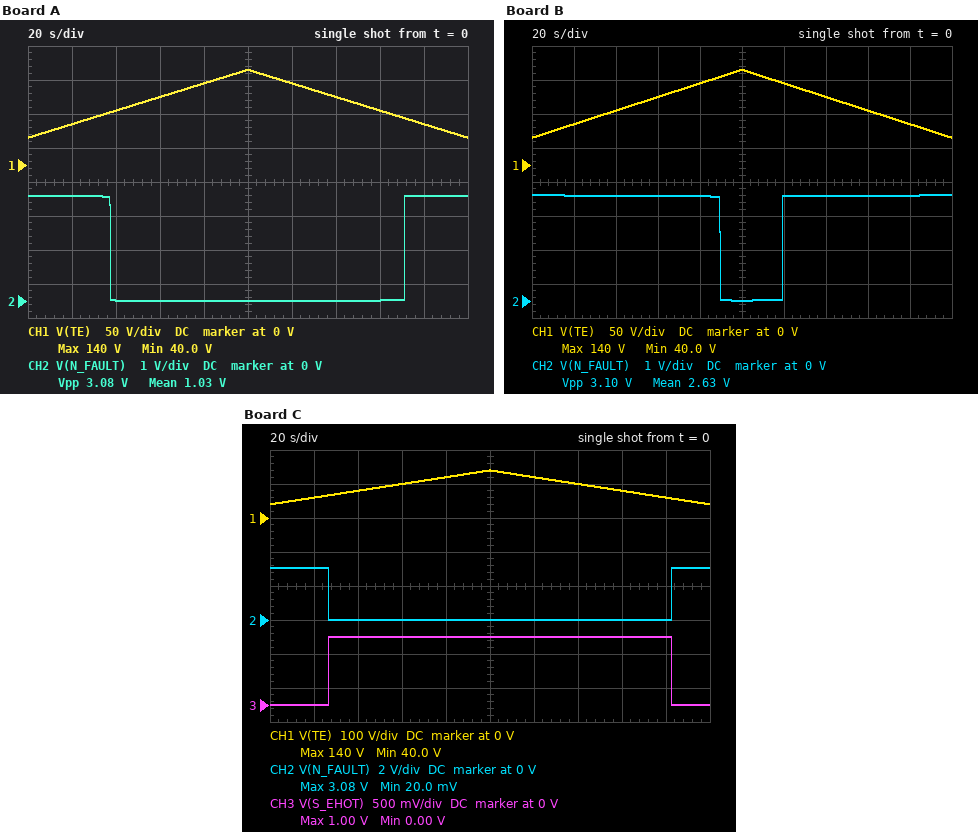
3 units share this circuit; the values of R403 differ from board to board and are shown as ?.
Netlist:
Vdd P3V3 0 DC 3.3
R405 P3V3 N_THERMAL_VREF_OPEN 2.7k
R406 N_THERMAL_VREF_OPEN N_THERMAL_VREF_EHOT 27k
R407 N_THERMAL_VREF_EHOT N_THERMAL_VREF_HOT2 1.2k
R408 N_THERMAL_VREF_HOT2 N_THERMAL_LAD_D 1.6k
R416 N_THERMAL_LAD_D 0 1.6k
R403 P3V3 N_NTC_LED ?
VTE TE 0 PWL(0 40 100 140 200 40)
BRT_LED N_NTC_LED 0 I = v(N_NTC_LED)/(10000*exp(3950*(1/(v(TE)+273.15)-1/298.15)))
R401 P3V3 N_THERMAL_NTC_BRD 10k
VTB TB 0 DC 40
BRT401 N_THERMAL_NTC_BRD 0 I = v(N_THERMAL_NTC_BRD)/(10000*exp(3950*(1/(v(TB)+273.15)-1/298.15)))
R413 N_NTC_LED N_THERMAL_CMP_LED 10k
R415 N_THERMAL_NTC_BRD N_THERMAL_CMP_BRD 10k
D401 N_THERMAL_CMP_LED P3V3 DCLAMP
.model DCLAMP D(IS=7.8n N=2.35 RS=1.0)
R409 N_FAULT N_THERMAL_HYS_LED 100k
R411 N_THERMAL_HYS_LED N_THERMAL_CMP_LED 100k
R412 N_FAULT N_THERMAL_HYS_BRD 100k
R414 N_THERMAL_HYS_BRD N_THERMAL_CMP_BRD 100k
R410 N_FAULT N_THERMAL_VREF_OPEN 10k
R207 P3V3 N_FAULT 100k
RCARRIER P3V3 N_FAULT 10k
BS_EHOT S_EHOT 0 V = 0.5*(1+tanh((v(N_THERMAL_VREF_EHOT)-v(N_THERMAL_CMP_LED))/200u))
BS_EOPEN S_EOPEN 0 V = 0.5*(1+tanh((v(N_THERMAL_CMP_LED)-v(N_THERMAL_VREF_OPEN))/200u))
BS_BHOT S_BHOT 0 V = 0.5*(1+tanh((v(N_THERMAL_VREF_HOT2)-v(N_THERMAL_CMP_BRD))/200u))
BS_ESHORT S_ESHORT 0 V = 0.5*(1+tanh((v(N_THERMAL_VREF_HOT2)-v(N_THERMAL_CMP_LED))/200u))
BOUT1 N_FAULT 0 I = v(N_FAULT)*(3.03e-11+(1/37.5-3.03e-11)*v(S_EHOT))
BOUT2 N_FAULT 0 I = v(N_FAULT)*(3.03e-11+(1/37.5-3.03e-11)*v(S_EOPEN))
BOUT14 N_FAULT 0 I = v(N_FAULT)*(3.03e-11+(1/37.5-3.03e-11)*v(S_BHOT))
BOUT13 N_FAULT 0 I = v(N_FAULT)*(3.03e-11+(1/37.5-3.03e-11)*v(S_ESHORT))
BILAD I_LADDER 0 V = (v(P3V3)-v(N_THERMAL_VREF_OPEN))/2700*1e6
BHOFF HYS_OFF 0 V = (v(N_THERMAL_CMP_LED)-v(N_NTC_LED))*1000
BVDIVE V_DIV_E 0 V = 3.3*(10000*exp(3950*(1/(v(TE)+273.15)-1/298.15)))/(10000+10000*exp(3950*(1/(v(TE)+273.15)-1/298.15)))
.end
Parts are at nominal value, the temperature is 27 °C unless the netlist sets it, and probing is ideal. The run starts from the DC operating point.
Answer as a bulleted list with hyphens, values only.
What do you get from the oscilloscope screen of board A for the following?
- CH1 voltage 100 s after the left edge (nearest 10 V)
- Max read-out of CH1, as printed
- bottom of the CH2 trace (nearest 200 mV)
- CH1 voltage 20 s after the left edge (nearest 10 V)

- 140 V
- 140 V
- 0 V
- 60 V
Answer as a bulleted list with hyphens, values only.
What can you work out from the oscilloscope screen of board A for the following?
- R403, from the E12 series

- 15 kΩ
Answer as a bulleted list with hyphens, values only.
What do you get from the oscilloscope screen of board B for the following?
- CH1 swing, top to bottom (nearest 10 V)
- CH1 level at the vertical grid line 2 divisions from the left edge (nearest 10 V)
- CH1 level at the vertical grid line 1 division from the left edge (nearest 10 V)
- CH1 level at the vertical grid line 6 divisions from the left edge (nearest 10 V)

- 100 V
- 80 V
- 60 V
- 120 V
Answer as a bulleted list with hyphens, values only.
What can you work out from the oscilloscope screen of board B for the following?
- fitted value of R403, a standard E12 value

- 3.3 kΩ
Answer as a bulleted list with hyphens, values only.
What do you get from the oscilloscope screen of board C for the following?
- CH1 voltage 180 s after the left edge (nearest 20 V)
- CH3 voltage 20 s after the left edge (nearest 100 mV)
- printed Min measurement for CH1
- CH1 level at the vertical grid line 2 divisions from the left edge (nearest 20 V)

- 60 V
- 0 V
- 40.0 V
- 80 V
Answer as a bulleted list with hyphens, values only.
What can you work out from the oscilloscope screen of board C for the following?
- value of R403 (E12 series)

- 22 kΩ
